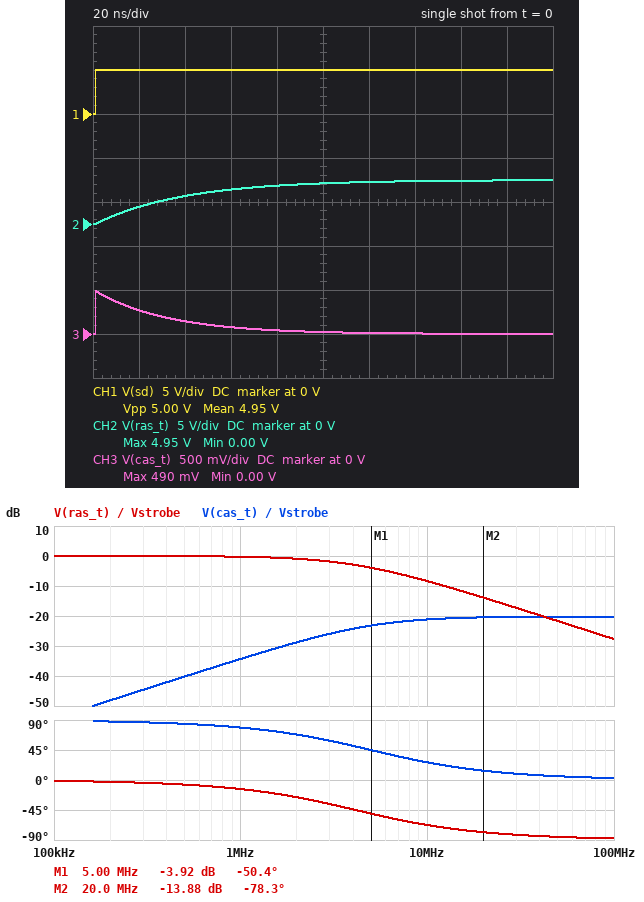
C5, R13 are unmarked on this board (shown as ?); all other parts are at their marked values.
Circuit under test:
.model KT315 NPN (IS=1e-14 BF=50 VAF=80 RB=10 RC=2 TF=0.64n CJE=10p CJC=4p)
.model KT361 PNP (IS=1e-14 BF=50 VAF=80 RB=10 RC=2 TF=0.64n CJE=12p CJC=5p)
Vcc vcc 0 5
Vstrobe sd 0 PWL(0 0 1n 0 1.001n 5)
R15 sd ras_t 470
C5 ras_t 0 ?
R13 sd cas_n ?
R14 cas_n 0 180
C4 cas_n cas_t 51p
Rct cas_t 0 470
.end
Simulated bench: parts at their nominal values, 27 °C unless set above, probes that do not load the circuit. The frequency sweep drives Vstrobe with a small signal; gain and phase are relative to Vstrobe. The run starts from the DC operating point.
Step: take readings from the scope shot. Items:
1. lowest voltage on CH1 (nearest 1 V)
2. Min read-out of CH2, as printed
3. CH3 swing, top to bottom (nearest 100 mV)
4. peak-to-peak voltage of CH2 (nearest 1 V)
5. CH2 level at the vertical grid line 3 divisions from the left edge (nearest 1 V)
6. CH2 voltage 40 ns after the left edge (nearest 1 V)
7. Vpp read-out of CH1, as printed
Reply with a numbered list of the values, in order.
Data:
1. 0 V
2. 0.00 V
3. 500 mV
4. 5 V
5. 4 V
6. 3 V
7. 5.00 V
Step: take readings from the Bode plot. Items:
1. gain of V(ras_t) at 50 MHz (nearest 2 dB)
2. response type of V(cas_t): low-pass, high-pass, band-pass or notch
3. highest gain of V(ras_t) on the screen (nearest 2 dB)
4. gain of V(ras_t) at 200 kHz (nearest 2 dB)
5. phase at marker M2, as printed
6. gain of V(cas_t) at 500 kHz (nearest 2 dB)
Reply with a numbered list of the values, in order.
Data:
1. -22 dB
2. high-pass
3. 0 dB
4. 0 dB
5. -78.3 deg
6. -40 dB
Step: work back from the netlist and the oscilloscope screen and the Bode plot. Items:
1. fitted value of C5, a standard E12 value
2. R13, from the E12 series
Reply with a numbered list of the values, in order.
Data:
1. 82 pF
2. 1.2 kΩ
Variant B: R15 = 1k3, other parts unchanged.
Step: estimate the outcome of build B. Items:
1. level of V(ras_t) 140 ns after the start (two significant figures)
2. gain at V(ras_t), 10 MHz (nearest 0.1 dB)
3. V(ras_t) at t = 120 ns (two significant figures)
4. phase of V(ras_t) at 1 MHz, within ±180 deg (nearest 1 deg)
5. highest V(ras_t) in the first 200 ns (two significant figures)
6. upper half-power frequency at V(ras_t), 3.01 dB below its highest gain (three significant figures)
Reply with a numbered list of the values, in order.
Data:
1. 3.6 V
2. -16.6 dB
3. 3.4 V
4. -34 deg
5. 4.2 V
6. 1.49 MHz
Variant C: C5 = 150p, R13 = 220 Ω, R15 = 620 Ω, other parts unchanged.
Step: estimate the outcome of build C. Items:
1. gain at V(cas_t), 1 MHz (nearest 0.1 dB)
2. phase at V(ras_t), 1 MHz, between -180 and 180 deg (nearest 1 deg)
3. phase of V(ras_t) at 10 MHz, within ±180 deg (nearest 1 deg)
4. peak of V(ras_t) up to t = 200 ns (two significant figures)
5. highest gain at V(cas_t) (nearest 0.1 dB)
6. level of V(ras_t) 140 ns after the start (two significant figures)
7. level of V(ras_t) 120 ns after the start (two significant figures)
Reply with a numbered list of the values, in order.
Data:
1. -23.5 dB
2. -30 deg
3. -80 deg
4. 4.4 V
5. -8.6 dB
6. 3.9 V
7. 3.6 V
